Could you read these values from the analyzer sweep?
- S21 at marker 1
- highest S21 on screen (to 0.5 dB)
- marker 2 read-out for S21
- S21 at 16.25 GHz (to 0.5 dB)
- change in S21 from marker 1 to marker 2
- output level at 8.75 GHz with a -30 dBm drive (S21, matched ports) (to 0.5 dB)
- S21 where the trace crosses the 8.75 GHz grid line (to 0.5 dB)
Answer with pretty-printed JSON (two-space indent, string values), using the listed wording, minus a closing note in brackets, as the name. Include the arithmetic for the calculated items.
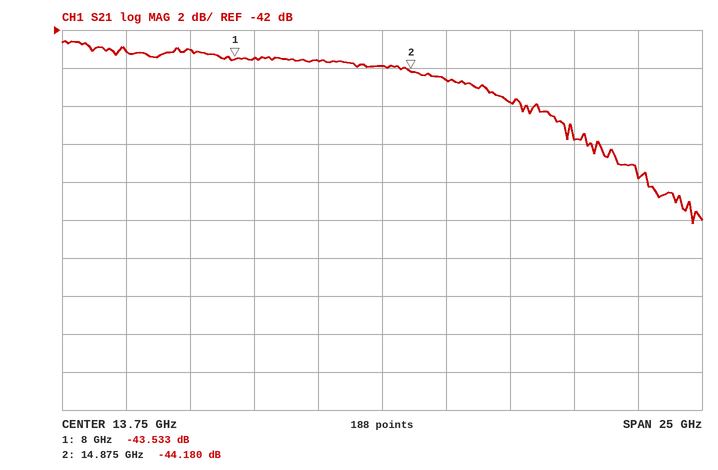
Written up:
{
  "S21 at marker 1": "-43.533 dB",
  "highest S21 on screen": "-42.5 dB",
  "marker 2 read-out for S21": "-44.180 dB",
  "S21 at 16.25 GHz": "-44.5 dB",
  "change in S21 from marker 1 to marker 2": "-44.18 − (-43.533) = -0.647 dB",
  "output level at 8.75 GHz with a -30 dBm drive (S21, matched ports)": "-30 dBm + (-43.5 dB) = -73.5 dBm",
  "S21 where the trace crosses the 8.75 GHz grid line": "-43.5 dB"
}
